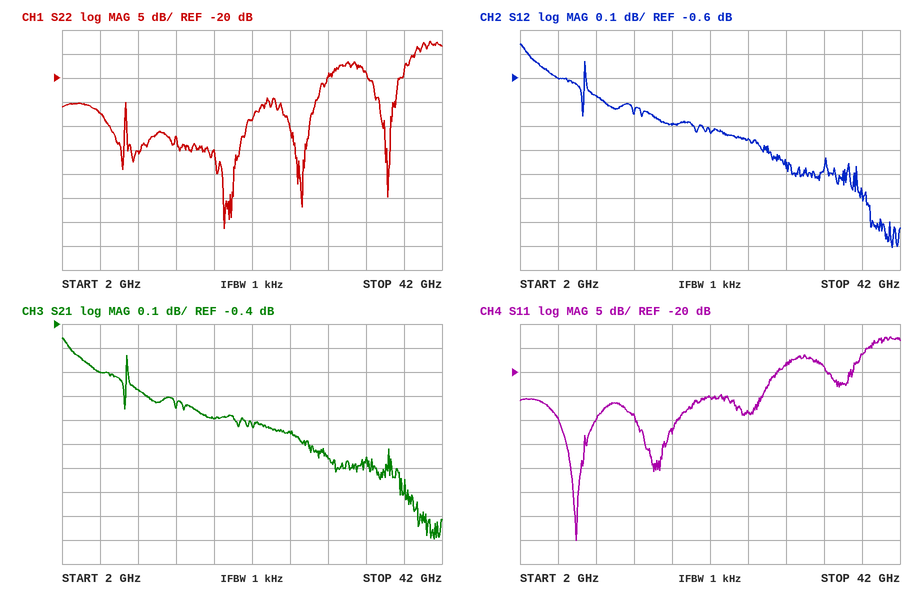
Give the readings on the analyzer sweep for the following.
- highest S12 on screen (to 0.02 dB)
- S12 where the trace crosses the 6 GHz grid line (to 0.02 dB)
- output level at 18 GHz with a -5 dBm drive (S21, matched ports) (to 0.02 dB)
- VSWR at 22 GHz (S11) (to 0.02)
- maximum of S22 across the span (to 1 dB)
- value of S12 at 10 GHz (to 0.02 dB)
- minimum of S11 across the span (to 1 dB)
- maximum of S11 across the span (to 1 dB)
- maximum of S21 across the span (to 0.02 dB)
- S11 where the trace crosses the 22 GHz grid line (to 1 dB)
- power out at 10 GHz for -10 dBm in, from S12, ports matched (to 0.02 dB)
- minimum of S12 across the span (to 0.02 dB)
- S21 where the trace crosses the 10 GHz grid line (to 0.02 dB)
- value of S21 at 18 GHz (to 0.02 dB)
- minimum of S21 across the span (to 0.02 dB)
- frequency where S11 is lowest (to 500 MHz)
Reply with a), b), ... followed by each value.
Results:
a) -0.46 dB
b) -0.60 dB
c) -5.80 dBm
d) 1.12
e) -12 dB
f) -0.68 dB
g) -55 dB
h) -13 dB
i) -0.46 dB
j) -25 dB
k) -10.68 dBm
l) -1.30 dB
m) -0.68 dB
n) -0.80 dB
o) -1.30 dB
p) 8.0 GHz
